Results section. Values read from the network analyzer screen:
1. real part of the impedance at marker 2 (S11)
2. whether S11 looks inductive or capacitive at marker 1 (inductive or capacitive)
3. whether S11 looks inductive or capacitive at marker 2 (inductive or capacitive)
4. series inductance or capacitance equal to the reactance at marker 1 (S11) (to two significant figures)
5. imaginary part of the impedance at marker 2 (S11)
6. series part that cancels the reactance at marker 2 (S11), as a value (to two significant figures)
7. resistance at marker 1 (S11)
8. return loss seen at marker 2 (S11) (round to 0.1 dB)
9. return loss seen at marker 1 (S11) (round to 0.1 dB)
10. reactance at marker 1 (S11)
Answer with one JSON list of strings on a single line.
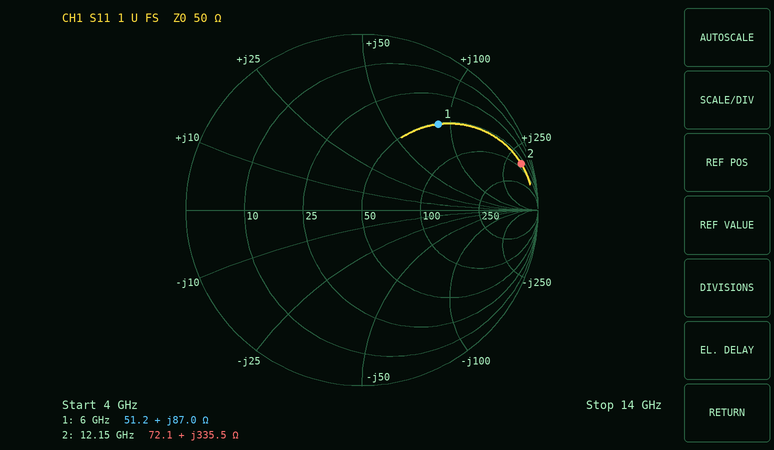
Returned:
["72.1 Ω", "inductive", "inductive", "2.3 nH", "+335.5 Ω", "39 fF", "51.2 Ω", "0.5 dB", "3.7 dB", "+87.0 Ω"]
